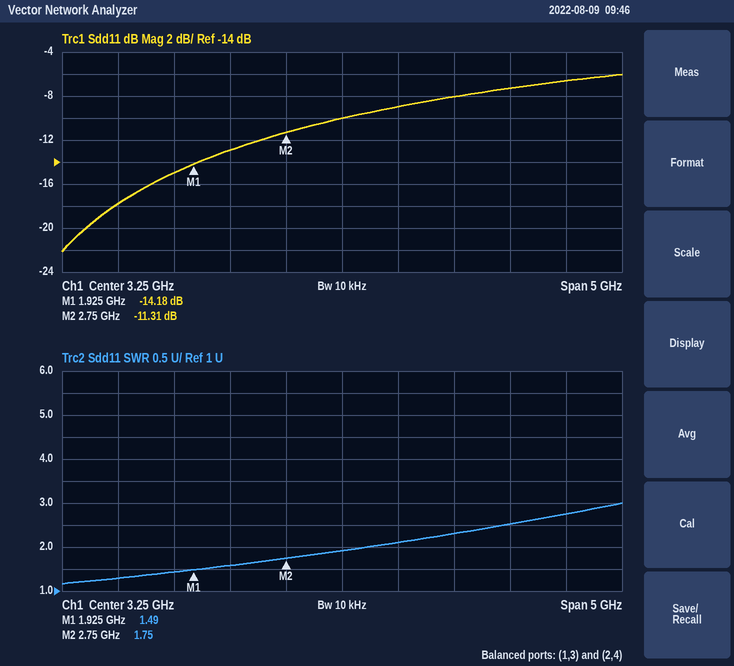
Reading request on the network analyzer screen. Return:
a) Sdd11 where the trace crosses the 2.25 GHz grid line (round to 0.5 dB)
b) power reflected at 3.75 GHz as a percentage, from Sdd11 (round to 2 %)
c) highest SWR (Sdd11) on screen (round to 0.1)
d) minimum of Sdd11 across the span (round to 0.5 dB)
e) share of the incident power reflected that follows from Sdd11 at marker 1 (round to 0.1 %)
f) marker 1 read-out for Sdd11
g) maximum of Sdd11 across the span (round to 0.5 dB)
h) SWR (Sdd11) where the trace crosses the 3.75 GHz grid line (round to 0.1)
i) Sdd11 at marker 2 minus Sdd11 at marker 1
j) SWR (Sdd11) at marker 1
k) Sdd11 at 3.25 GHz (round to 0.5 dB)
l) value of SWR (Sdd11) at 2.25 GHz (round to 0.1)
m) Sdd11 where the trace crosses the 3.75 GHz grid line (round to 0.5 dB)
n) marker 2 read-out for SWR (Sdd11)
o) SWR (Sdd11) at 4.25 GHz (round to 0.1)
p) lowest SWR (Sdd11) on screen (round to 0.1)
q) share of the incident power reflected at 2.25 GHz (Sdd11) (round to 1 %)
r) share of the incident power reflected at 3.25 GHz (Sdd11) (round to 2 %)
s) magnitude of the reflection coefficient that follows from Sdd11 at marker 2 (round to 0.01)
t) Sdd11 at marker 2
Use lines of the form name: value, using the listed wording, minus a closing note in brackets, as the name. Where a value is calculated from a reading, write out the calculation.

Sdd11 where the trace crosses the 2.25 GHz grid line: -13.0 dB
power reflected at 3.75 GHz as a percentage, from Sdd11: 10^(-9/10) ≈ 12.6 %, so 12 % to the nearest 2 %
highest SWR (Sdd11) on screen: 3.0
minimum of Sdd11 across the span: -22.0 dB
share of the incident power reflected that follows from Sdd11 at marker 1: 10^(-14.18/10) ≈ 3.8 %
marker 1 read-out for Sdd11: -14.18 dB
maximum of Sdd11 across the span: -6.0 dB
SWR (Sdd11) where the trace crosses the 3.75 GHz grid line: 2.1
Sdd11 at marker 2 minus Sdd11 at marker 1: -11.31 − (-14.18) = 2.87 dB
SWR (Sdd11) at marker 1: 1.49
Sdd11 at 3.25 GHz: -10.0 dB
value of SWR (Sdd11) at 2.25 GHz: 1.6
Sdd11 where the trace crosses the 3.75 GHz grid line: -9.0 dB
marker 2 read-out for SWR: 1.75
SWR (Sdd11) at 4.25 GHz: 2.3
lowest SWR (Sdd11) on screen: 1.2
share of the incident power reflected at 2.25 GHz (Sdd11): 10^(-13/10) ≈ 5 %
share of the incident power reflected at 3.25 GHz (Sdd11): 10^(-10/10) ≈ 10 %
magnitude of the reflection coefficient that follows from Sdd11 at marker 2: 10^(-11.31/20) ≈ 0.27
Sdd11 at marker 2: -11.31 dB
